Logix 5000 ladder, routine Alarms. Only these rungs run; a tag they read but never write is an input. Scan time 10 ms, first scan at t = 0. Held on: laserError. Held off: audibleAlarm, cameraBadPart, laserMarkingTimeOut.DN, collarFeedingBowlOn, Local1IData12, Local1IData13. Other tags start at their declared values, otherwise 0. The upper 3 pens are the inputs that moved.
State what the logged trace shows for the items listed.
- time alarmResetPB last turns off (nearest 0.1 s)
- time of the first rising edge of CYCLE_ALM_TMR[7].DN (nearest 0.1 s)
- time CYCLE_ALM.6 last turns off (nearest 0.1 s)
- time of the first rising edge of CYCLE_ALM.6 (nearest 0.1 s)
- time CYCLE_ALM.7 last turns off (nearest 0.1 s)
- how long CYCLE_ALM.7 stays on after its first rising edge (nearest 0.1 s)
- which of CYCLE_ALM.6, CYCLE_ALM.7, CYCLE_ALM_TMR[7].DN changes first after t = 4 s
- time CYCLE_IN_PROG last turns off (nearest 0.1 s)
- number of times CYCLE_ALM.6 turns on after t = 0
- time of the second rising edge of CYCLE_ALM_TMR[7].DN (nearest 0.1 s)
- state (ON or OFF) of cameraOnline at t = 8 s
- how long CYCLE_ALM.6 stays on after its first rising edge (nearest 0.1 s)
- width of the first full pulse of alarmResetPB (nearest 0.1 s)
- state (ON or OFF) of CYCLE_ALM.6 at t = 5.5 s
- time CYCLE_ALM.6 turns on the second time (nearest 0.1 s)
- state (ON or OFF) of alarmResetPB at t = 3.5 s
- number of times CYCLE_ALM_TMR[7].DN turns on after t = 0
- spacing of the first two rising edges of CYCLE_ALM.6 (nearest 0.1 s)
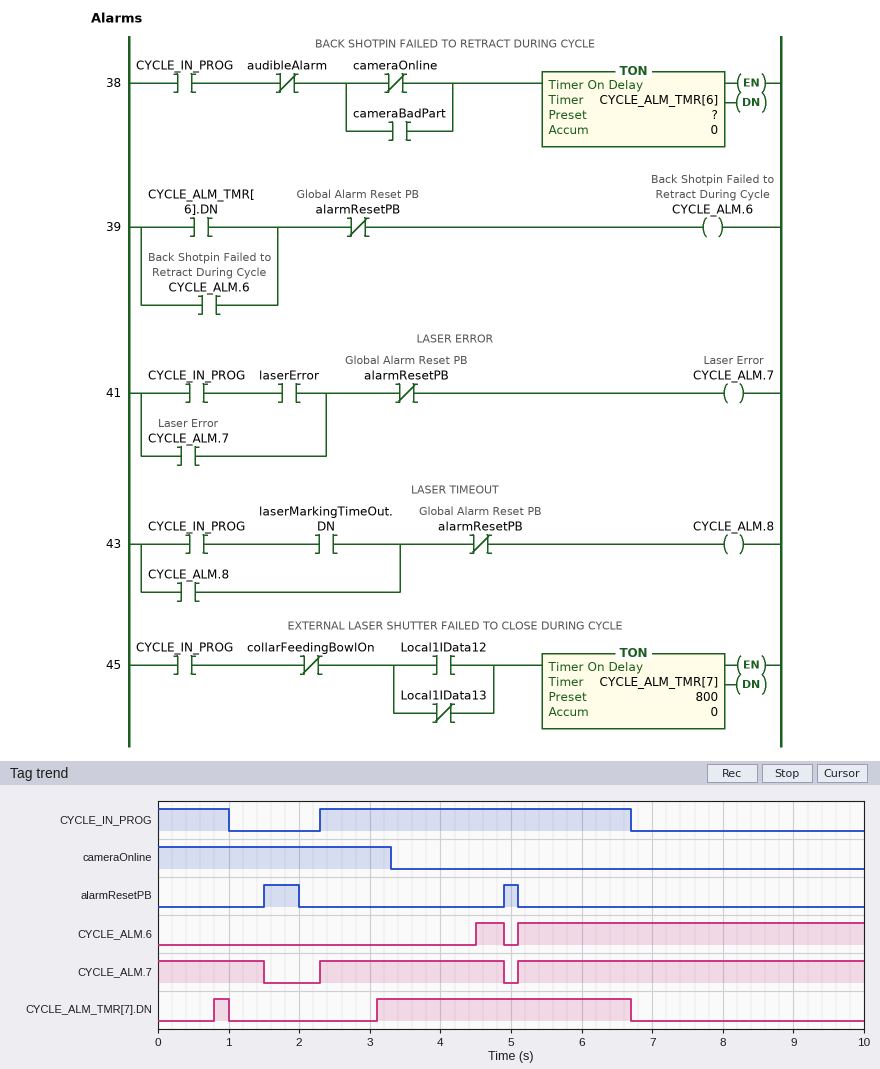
5.1 s
0.8 s
4.9 s
4.5 s
4.9 s
2.6 s
CYCLE_ALM.6
6.7 s
2
3.1 s
OFF
0.4 s
0.5 s
ON
5.1 s
OFF
2
0.6 s
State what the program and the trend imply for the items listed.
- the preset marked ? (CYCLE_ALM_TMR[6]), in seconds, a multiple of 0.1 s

1.2 s
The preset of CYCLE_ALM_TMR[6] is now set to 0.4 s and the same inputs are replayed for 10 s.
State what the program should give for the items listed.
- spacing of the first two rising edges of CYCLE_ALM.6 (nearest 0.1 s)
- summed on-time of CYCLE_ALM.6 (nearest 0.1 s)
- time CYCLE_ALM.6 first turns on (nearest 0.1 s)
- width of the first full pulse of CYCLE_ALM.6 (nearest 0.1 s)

1.4 s
6.1 s
3.7 s
1.2 s
